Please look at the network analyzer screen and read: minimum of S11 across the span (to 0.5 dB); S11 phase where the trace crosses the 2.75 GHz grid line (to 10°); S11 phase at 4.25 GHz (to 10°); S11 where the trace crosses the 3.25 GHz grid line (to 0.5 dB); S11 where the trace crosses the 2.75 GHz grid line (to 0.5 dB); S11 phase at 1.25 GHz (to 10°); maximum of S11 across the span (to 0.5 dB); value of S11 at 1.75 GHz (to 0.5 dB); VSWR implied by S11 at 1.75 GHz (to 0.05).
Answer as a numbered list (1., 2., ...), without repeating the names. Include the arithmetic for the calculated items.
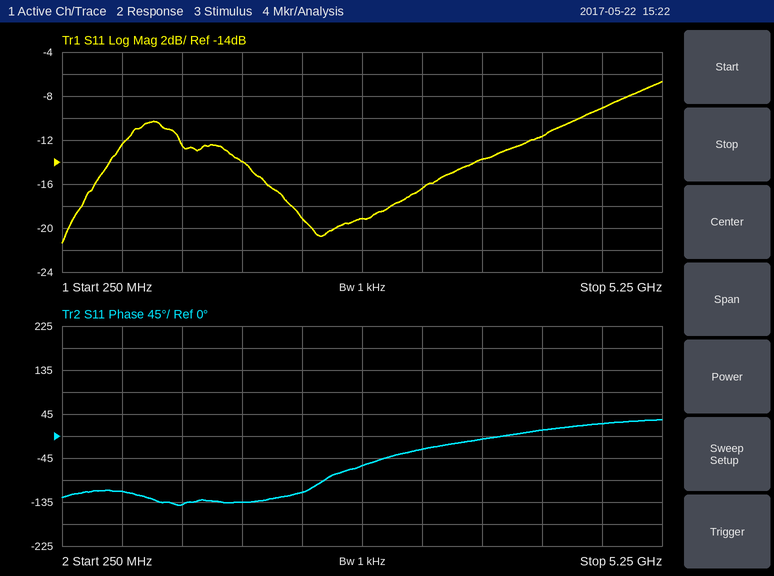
1. -21.5 dB
2. -60°
3. 10°
4. -16.5 dB
5. -19.0 dB
6. -140°
7. -6.5 dB
8. -14.0 dB
9. |Γ| = 10^(-14/20) = 0.1995; VSWR = (1 + 0.1995)/(1 − 0.1995) ≈ 1.50
